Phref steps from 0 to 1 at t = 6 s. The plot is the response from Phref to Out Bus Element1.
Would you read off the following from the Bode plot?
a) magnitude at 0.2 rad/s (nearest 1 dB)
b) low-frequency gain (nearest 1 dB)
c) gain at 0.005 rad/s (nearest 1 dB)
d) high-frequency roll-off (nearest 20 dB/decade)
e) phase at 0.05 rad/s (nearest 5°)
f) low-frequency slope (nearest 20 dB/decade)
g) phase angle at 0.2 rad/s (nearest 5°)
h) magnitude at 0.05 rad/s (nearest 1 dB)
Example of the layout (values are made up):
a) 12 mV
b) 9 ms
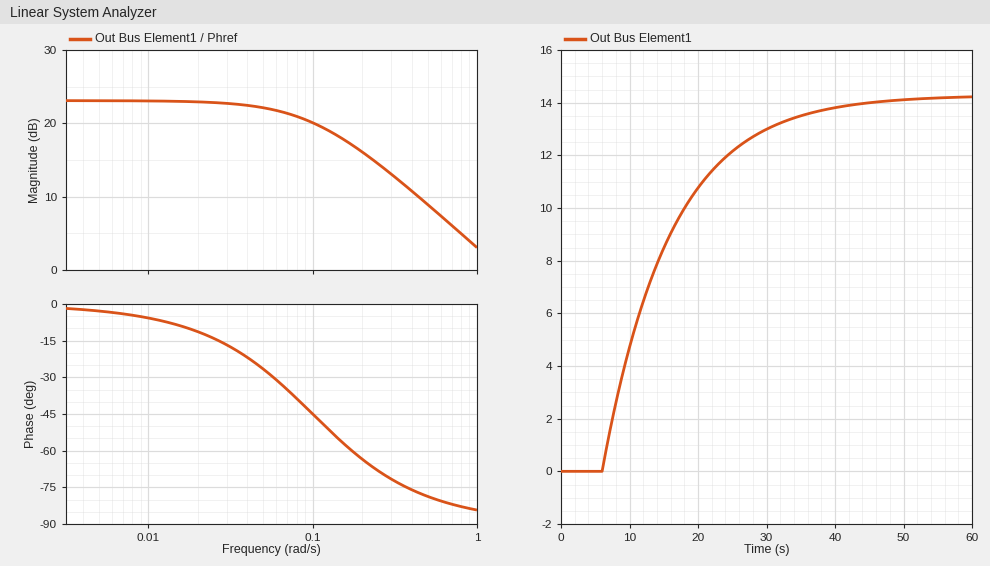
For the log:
a) 16 dB
b) 23 dB
c) 23 dB
d) -20 dB/decade
e) -25°
f) 0 dB/decade
g) -65°
h) 22 dB
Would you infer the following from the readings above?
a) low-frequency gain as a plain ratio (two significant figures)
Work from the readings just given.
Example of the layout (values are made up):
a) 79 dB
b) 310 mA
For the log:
a) 14
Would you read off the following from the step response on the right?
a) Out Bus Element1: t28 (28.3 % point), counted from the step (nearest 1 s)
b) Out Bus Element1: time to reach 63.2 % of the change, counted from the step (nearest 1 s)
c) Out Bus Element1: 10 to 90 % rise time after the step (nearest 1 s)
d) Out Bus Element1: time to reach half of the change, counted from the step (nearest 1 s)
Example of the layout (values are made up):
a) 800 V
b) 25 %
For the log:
a) 3 s
b) 10 s
c) 22 s
d) 7 s
